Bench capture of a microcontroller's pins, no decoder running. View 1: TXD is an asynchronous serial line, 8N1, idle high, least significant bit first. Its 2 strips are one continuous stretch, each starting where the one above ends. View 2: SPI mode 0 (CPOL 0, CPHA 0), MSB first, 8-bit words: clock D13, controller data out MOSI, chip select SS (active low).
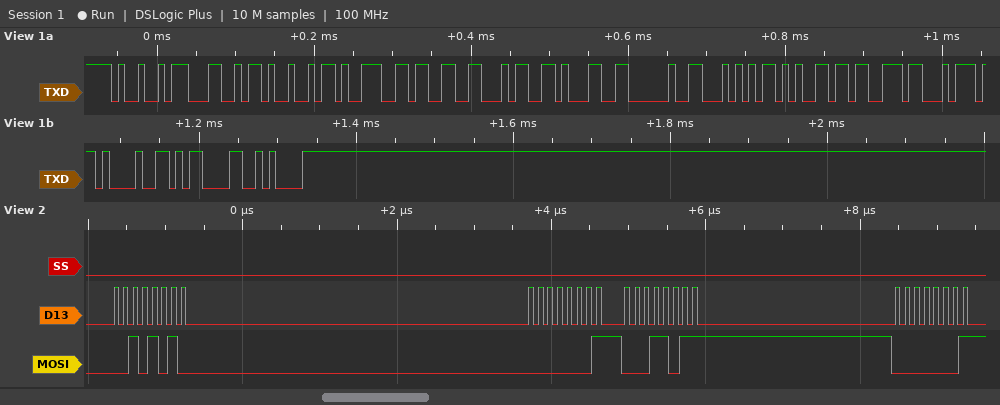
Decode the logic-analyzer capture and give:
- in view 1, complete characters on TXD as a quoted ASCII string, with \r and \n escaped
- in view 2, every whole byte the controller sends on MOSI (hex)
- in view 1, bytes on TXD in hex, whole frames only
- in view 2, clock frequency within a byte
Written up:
"ILI9341 Test!\r\n"
2A 01 1B 01
49 4C 49 39 33 34 31 20 54 65 73 74 21 0D 0A
8 MHz
